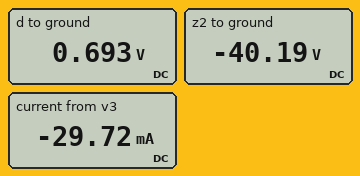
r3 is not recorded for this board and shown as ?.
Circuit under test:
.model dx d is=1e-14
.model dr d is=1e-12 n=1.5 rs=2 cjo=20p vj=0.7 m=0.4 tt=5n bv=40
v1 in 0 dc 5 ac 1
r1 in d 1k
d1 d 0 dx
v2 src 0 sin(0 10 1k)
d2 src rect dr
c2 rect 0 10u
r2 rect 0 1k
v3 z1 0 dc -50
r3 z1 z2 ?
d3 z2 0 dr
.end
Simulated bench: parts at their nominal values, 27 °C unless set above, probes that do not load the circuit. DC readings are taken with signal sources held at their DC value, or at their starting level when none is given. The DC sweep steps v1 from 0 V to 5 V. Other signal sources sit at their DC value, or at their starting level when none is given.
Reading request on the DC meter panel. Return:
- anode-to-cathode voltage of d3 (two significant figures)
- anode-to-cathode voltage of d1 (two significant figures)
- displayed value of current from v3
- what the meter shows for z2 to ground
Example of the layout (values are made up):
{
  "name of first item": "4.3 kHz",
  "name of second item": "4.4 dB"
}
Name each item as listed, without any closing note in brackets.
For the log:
{
  "anode-to-cathode voltage of d3": "-40 V",
  "anode-to-cathode voltage of d1": "690 mV",
  "displayed value of current from v3": "-29.72 mA",
  "what the meter shows for z2 to ground": "-40.19 V"
}
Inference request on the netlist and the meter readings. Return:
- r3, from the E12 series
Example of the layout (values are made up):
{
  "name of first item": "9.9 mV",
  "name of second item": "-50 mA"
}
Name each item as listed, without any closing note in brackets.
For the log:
{
  "r3, from the E12 series": "330 Ω"
}
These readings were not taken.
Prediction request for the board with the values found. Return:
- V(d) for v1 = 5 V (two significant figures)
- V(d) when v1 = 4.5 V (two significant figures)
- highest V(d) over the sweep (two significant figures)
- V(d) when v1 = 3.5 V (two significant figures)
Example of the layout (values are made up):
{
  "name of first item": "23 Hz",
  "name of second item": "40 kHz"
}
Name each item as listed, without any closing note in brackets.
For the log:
{
  "V(d) for v1 = 5 V": "690 mV",
  "V(d) when v1 = 4.5 V": "690 mV",
  "highest V(d) over the sweep": "690 mV",
  "V(d) when v1 = 3.5 V": "680 mV"
}
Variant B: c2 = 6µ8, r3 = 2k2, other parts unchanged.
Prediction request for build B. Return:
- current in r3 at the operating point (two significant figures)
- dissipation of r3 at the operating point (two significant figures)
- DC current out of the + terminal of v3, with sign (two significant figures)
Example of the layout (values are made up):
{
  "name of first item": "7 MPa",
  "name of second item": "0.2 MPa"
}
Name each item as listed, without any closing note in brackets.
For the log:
{
  "current in r3 at the operating point": "4.5 mA",
  "dissipation of r3 at the operating point": "45 mW",
  "DC current out of the + terminal of v3, with sign": "-4.5 mA"
}
